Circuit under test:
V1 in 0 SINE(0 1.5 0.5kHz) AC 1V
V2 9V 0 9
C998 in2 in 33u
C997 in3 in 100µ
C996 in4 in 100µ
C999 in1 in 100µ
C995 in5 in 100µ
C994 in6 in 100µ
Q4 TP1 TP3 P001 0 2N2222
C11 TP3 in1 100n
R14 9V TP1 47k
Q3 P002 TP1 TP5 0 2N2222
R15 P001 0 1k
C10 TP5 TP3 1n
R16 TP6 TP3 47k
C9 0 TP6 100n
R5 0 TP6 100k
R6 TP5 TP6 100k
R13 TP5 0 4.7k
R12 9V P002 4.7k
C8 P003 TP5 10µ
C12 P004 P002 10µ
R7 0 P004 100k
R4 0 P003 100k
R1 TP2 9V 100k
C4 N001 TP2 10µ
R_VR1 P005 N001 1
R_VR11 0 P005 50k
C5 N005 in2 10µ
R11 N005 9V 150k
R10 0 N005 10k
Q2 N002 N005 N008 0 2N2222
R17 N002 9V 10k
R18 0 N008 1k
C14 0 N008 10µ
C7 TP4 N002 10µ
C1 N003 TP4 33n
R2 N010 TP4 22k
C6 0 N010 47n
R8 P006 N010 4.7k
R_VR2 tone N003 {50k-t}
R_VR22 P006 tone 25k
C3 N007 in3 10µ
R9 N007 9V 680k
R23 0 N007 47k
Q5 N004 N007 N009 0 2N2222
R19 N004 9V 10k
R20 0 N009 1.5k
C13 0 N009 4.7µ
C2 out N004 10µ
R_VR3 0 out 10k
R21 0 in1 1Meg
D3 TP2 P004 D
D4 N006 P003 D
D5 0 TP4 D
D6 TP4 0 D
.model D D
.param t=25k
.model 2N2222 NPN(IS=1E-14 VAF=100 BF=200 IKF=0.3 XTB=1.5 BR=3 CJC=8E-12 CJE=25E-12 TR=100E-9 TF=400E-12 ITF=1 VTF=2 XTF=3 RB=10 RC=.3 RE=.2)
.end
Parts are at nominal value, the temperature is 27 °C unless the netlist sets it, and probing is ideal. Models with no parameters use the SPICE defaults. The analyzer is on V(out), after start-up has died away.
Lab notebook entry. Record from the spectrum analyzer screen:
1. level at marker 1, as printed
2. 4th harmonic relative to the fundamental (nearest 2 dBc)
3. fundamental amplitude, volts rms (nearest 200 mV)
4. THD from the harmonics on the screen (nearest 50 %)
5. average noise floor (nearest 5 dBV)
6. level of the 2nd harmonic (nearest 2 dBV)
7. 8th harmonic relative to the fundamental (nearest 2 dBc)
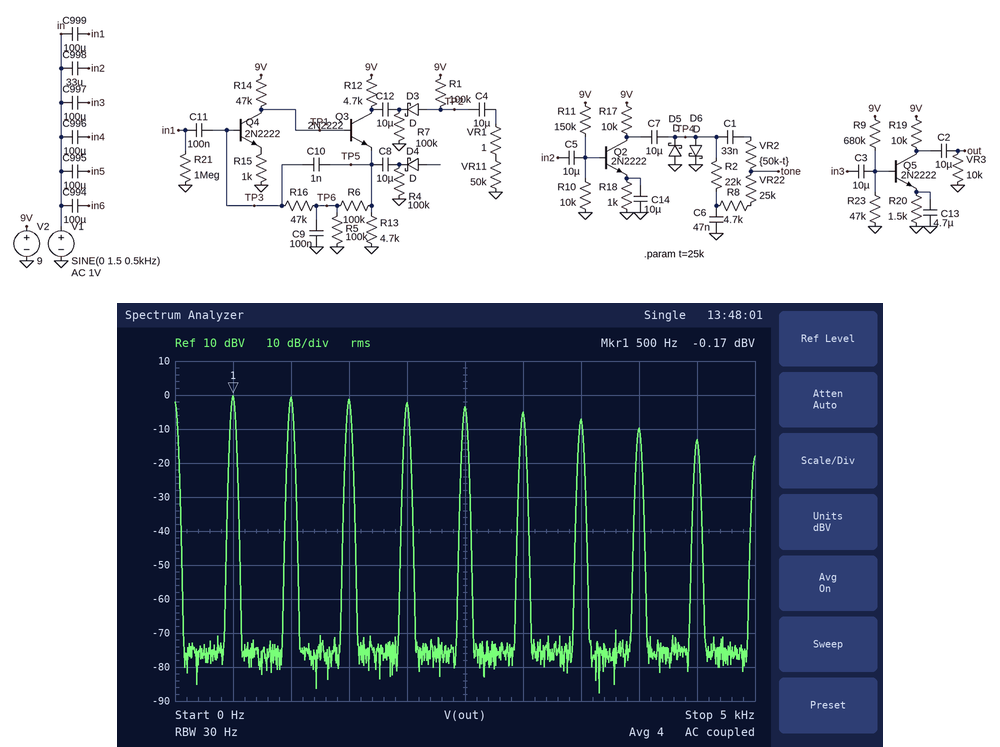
-0.17 dBV
-2 dBc
1.0 V
200 %
-75 dBV
0 dBV
-10 dBc
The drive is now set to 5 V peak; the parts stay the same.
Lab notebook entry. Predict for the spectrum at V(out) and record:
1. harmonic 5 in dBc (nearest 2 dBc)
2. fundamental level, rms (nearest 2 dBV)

-2 dBc
-2 dBV
